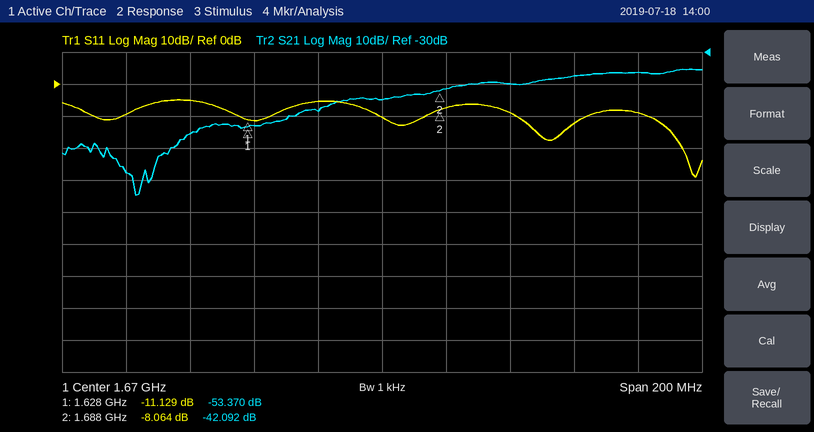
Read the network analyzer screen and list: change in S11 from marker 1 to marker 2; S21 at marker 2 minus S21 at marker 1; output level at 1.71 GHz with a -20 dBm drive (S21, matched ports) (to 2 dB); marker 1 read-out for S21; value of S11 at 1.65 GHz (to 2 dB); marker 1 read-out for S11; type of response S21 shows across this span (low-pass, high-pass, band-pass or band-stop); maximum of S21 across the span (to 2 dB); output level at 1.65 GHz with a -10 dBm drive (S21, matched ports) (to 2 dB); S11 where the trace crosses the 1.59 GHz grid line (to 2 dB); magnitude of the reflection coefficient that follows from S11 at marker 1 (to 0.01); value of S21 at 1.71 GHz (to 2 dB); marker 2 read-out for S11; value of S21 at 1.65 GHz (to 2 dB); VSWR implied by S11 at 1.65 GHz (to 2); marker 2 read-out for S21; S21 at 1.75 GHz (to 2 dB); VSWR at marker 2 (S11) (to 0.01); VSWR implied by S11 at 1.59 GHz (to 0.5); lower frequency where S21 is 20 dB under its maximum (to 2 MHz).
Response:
3.065 dB
11.278 dB
-60 dBm
-53.370 dB
-6 dB
-11.129 dB
high-pass
-36 dB
-58 dBm
-10 dB
0.28
-40 dB
-8.064 dB
-48 dB
4
-42.092 dB
-36 dB
2.31
2.0
1.610 GHz
